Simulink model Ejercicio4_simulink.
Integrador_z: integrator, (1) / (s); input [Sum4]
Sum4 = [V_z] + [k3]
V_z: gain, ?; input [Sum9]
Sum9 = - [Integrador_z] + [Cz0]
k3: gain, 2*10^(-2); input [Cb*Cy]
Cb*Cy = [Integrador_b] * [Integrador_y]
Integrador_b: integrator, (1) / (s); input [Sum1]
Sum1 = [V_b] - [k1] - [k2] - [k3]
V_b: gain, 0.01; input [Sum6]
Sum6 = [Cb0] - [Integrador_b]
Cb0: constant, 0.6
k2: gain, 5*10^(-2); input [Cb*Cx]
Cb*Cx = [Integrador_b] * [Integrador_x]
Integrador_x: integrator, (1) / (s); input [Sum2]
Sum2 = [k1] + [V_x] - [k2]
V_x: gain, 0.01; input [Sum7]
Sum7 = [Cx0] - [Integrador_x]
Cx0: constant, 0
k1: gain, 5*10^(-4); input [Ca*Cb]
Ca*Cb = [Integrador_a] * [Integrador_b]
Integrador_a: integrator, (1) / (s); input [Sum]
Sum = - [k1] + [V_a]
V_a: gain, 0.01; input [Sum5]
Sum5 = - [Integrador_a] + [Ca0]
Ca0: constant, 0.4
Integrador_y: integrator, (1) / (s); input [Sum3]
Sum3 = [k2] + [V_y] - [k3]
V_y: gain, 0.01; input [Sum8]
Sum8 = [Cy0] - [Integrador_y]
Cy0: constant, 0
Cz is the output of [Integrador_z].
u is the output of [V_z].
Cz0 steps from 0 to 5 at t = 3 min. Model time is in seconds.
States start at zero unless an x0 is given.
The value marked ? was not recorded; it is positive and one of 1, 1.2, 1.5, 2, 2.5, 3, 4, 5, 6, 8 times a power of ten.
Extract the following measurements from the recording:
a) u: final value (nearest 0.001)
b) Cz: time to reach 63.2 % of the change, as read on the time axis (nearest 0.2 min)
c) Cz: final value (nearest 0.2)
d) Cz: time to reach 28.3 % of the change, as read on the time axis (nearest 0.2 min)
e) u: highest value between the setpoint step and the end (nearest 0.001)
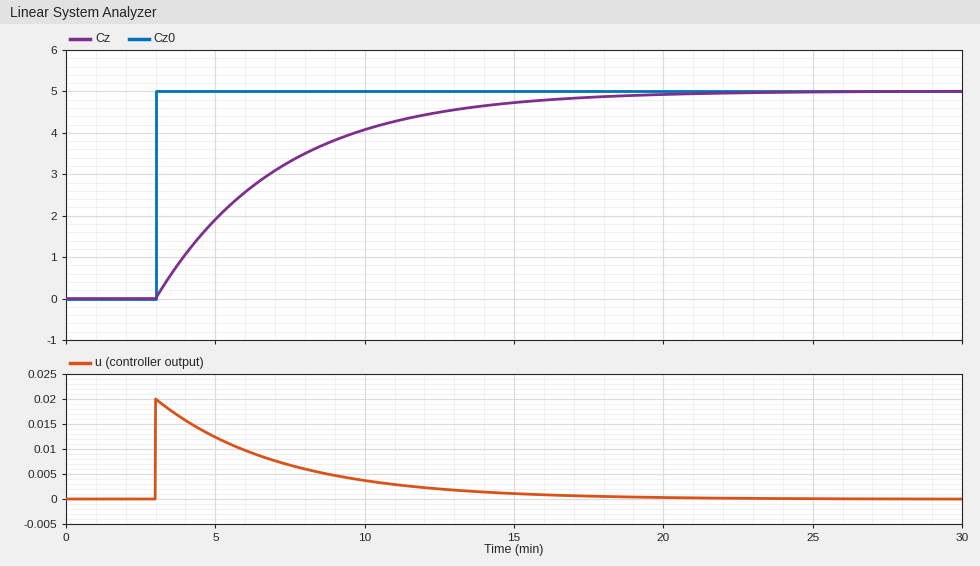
0.000
7.2 min
5.0
4.4 min
0.020
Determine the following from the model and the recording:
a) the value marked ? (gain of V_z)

0.004
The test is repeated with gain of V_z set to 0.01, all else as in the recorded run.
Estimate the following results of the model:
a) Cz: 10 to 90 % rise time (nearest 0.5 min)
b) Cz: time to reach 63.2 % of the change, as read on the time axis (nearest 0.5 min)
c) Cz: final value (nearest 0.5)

3.5 min
4.5 min
5.0
